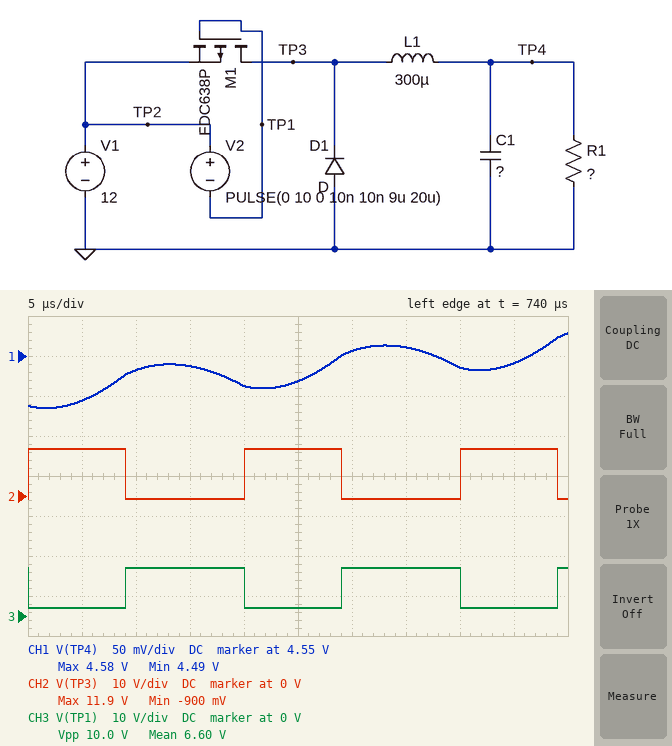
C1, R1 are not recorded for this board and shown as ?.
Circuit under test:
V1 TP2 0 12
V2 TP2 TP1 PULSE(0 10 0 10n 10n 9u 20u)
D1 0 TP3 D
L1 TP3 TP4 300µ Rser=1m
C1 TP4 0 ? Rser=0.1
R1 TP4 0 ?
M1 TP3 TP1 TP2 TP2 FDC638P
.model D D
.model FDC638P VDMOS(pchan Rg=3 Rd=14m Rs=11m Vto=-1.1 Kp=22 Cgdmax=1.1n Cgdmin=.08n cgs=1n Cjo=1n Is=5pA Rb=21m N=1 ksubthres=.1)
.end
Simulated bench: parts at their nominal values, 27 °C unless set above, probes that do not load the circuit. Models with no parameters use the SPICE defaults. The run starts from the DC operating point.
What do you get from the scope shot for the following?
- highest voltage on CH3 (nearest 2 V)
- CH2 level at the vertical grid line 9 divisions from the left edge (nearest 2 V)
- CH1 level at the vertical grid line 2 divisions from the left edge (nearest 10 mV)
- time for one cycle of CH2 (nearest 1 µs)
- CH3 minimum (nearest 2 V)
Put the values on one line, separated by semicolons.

12 V; 12 V; 4.53 V; 20 µs; 2 V
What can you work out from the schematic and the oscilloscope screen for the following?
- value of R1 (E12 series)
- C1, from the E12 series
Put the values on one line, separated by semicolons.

1 Ω; 12 µF
